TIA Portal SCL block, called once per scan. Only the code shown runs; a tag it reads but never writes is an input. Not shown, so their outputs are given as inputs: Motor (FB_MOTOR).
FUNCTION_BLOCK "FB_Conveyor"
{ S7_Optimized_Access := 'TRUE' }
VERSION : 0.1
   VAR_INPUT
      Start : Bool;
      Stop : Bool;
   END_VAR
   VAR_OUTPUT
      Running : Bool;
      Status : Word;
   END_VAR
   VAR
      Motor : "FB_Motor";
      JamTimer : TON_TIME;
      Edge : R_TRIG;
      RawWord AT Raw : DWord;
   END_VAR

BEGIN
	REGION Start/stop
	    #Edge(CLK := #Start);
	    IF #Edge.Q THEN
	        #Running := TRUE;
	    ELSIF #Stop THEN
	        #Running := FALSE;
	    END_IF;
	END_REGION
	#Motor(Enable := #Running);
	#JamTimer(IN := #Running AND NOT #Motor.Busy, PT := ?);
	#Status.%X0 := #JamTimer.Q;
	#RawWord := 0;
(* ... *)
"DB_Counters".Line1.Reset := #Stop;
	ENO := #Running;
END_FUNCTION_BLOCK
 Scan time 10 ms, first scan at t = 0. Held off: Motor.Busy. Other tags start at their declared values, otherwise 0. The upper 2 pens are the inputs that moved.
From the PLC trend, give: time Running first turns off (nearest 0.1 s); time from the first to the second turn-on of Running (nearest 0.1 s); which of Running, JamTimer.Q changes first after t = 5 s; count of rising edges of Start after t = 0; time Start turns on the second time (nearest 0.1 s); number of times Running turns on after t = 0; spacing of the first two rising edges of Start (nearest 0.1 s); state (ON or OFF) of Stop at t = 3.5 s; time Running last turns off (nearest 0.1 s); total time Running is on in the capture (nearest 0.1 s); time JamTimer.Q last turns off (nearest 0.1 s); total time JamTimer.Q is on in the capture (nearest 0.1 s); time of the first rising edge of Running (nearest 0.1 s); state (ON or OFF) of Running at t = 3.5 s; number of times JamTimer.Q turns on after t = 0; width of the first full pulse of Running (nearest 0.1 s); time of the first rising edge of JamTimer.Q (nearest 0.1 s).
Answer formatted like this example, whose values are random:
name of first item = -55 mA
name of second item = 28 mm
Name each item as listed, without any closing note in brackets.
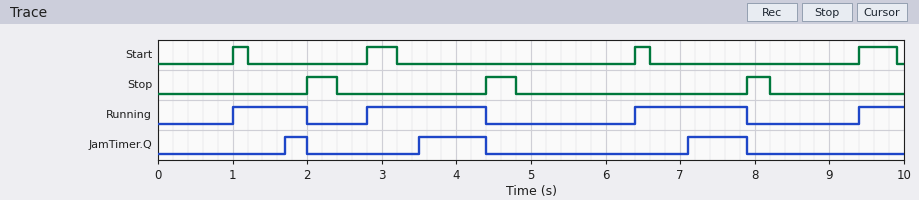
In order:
time Running first turns off = 2.0 s
time from the first to the second turn-on of Running = 1.8 s
which of Running, JamTimer.Q changes first after t = 5 s = Running
count of rising edges of Start after t = 0 = 4
time Start turns on the second time = 2.8 s
number of times Running turns on after t = 0 = 4
spacing of the first two rising edges of Start = 1.8 s
state (ON or OFF) of Stop at t = 3.5 s = OFF
time Running last turns off = 7.9 s
total time Running is on in the capture = 4.7 s
time JamTimer.Q last turns off = 7.9 s
total time JamTimer.Q is on in the capture = 2.0 s
time of the first rising edge of Running = 1.0 s
state (ON or OFF) of Running at t = 3.5 s = ON
number of times JamTimer.Q turns on after t = 0 = 3
width of the first full pulse of Running = 1.0 s
time of the first rising edge of JamTimer.Q = 1.7 s
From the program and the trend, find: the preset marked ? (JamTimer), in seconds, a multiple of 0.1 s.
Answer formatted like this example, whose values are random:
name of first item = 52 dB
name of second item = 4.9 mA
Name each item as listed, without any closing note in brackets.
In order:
the preset marked ? (JamTimer), in seconds, a multiple of 0.1 s = 0.7 s
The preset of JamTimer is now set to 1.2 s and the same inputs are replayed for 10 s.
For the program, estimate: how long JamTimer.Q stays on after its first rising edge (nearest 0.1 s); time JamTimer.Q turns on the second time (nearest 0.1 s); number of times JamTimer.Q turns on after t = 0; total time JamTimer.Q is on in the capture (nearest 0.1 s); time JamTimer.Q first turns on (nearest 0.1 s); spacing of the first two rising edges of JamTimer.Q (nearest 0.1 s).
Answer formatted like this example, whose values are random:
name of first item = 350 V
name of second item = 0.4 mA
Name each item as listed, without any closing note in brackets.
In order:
how long JamTimer.Q stays on after its first rising edge = 0.4 s
time JamTimer.Q turns on the second time = 7.6 s
number of times JamTimer.Q turns on after t = 0 = 2
total time JamTimer.Q is on in the capture = 0.7 s
time JamTimer.Q first turns on = 4.0 s
spacing of the first two rising edges of JamTimer.Q = 3.6 s
